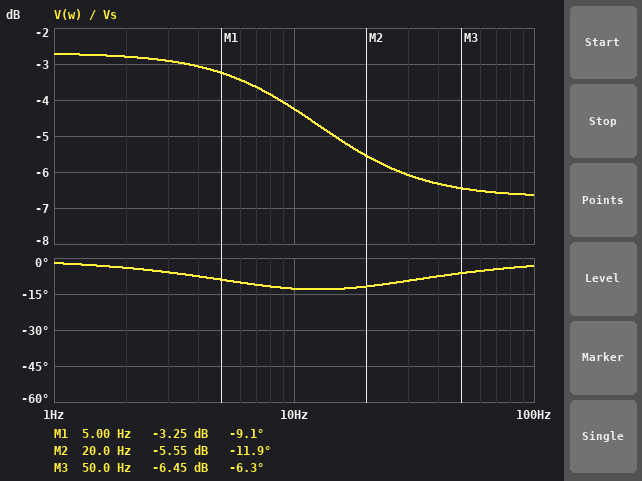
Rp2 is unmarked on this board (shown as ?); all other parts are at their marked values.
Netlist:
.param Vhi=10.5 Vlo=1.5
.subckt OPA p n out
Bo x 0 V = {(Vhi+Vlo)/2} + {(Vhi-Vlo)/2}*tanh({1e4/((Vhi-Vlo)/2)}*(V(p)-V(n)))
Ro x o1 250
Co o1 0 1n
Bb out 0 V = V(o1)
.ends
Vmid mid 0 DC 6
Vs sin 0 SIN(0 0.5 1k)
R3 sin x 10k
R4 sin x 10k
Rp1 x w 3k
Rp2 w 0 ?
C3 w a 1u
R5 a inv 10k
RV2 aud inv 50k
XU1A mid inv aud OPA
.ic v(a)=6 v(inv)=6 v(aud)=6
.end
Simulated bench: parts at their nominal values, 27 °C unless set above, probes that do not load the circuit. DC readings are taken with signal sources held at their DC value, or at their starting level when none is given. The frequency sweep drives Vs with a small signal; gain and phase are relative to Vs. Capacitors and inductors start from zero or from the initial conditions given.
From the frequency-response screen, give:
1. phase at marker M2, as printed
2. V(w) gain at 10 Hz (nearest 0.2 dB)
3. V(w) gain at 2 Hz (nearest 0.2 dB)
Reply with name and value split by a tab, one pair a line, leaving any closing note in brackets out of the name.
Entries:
phase at marker M2, as printed	-11.9 deg
V(w) gain at 10 Hz	-4.2 dB
V(w) gain at 2 Hz	-2.8 dB
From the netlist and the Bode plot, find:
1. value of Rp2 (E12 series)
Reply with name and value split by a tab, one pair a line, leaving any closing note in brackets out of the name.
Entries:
value of Rp2	22 kΩ
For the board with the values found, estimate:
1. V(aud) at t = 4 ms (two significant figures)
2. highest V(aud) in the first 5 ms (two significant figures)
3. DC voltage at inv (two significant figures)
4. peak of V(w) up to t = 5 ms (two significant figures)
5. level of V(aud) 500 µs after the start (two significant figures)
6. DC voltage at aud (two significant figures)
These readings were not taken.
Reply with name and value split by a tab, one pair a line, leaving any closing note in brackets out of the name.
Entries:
V(aud) at t = 4 ms	6.0 V
highest V(aud) in the first 5 ms	7.2 V
DC voltage at inv	6.0 V
peak of V(w) up to t = 5 ms	230 mV
level of V(aud) 500 µs after the start	6.0 V
DC voltage at aud	6.0 V
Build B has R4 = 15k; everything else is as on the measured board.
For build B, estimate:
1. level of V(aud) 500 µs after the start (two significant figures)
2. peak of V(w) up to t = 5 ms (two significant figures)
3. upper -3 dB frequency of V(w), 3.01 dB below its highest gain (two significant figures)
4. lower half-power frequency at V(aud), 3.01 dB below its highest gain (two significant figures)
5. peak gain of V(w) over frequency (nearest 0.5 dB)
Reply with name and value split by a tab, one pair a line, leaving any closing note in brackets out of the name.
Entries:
level of V(aud) 500 µs after the start	6.0 V
peak of V(w) up to t = 5 ms	220 mV
upper -3 dB frequency of V(w), 3.01 dB below its highest gain	19 Hz
lower half-power frequency at V(aud), 3.01 dB below its highest gain	9.7 Hz
peak gain of V(w) over frequency	-3.0 dB
